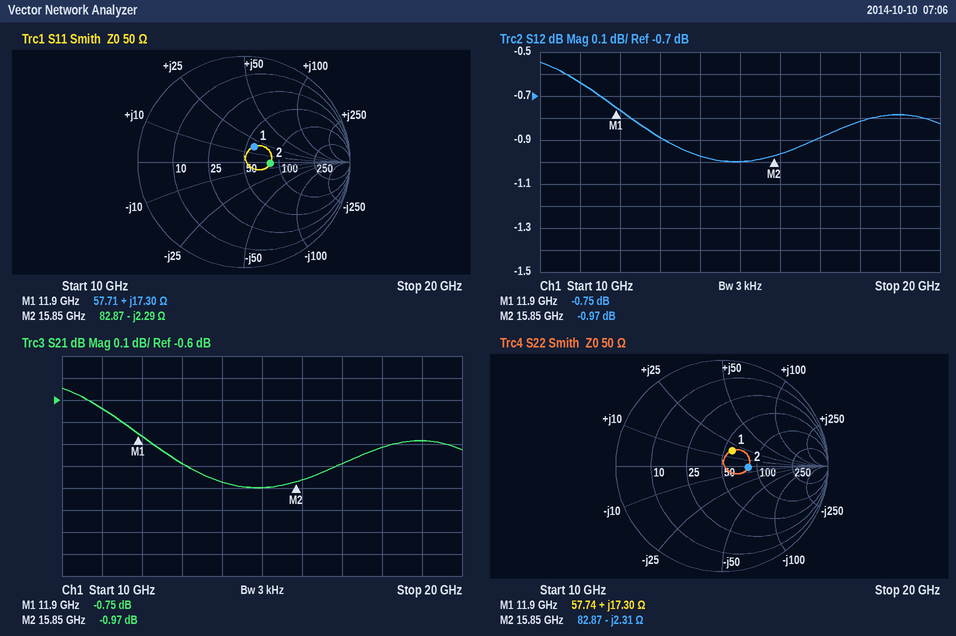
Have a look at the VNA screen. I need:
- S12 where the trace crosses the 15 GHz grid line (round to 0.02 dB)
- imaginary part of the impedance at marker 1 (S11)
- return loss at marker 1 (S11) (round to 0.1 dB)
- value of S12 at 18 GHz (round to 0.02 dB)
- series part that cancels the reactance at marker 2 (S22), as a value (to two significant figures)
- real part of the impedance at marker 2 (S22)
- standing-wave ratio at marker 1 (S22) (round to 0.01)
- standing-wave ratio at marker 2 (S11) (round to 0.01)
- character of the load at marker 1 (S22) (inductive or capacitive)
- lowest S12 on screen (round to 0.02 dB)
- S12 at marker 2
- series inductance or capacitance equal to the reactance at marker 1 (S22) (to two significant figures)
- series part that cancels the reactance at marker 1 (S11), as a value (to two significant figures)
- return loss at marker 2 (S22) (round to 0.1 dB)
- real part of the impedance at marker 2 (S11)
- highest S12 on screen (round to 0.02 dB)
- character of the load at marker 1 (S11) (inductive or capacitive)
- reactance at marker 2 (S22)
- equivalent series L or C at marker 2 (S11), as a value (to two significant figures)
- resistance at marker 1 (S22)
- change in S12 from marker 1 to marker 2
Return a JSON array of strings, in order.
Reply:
["-1.00 dB", "+17.30 Ω", "15.2 dB", "-0.82 dB", "23 pH", "82.87 Ω", "1.42", "1.66", "inductive", "-1.00 dB", "-0.97 dB", "230 pH", "770 fF", "12.1 dB", "82.87 Ω", "-0.54 dB", "inductive", "-2.31 Ω", "4.4 pF", "57.74 Ω", "-0.22 dB"]
